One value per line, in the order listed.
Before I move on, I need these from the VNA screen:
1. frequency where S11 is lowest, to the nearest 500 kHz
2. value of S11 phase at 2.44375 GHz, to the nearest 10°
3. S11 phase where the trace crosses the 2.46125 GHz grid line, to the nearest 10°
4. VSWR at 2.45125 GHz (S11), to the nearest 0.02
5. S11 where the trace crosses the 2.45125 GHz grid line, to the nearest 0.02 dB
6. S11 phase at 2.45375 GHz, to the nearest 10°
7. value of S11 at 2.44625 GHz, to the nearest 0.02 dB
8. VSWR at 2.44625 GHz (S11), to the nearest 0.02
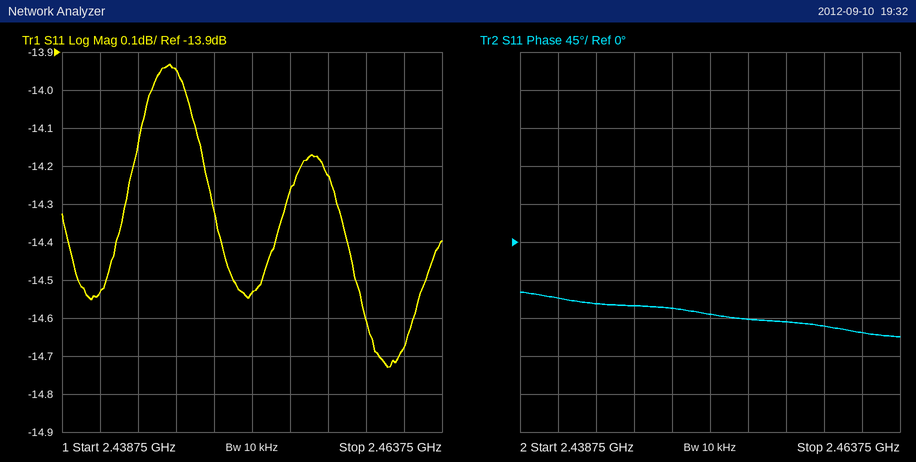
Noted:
2.4600 GHz
-70°
-110°
1.46
-14.54 dB
-90°
-13.94 dB
1.50
